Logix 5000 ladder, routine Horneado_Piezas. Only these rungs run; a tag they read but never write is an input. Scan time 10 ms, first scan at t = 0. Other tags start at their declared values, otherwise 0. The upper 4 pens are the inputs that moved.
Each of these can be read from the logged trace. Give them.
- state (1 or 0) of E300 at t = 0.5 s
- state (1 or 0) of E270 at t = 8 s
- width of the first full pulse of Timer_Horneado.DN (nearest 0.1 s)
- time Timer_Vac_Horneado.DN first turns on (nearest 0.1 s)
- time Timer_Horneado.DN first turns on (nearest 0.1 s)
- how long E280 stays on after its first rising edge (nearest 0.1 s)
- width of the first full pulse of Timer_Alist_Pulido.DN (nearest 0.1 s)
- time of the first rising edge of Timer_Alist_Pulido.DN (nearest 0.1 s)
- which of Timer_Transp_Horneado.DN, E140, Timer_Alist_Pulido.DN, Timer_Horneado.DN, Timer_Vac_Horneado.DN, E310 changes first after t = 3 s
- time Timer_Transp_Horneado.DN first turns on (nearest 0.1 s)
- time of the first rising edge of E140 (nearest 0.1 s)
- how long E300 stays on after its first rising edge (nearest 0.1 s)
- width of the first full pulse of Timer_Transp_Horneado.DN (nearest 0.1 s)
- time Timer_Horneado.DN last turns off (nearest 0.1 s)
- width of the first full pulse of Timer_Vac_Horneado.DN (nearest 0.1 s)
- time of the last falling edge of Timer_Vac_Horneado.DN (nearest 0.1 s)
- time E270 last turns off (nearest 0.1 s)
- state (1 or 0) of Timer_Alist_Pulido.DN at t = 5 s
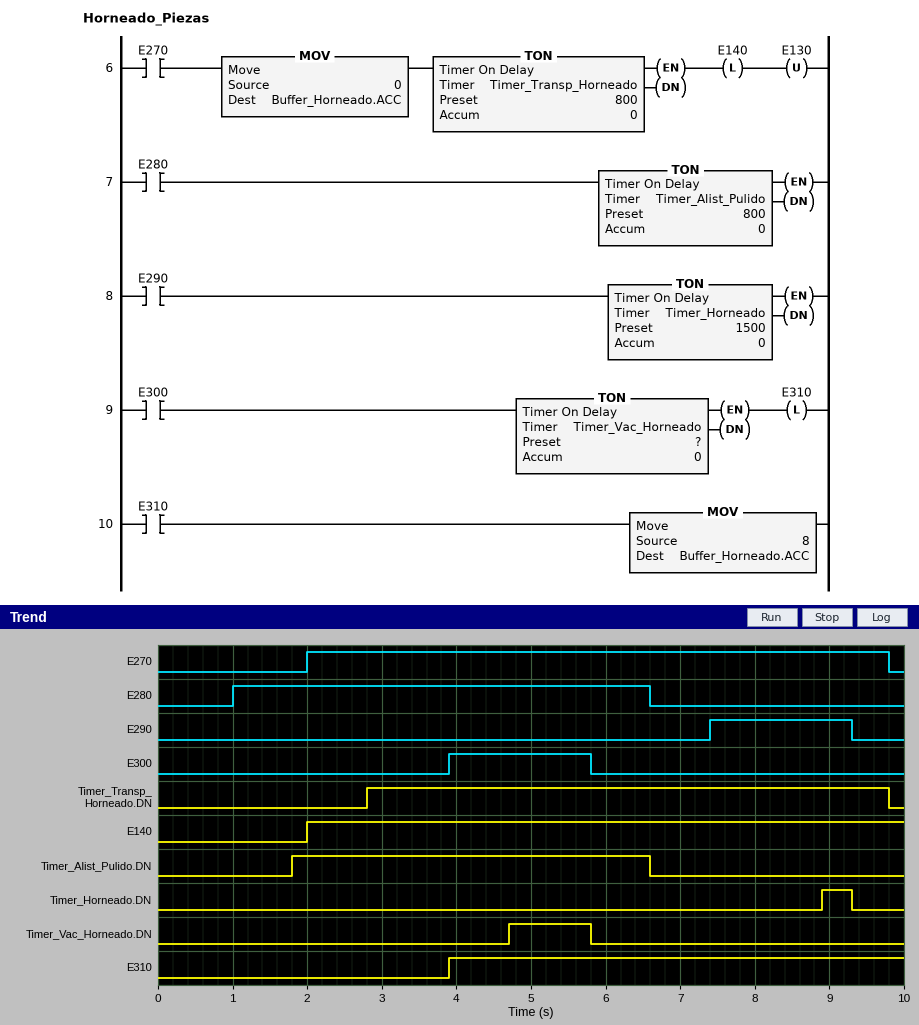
0
1
0.4 s
4.7 s
8.9 s
5.6 s
4.8 s
1.8 s
E310
2.8 s
2.0 s
1.9 s
7.0 s
9.3 s
1.1 s
5.8 s
9.8 s
1
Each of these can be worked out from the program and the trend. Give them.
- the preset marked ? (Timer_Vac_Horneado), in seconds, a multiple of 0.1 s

0.8 s
